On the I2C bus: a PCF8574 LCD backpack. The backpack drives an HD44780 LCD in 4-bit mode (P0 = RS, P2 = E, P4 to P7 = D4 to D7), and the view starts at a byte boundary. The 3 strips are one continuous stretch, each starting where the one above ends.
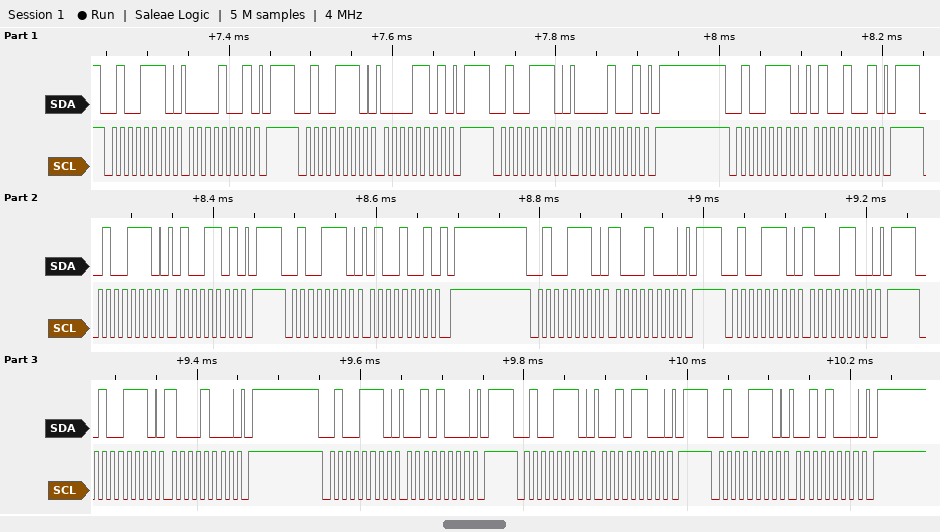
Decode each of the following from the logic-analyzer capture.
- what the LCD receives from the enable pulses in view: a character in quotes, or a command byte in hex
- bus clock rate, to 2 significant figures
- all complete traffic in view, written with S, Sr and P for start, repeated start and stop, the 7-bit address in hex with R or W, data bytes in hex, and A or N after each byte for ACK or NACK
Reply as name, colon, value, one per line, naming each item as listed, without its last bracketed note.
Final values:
what the LCD receives from the enable pulses in view: a character in quotes, or a command byte in hex: data 0x04 0x82
bus clock rate, to 2 significant figures: 100 kHz
all complete traffic in view, written with S, Sr and P for start, repeated start and stop, the 7-bit address in hex with R or W, data bytes in hex, and A or N after each byte for ACK or NACK: S 27W A 09 A P S 27W A 0D A P S 27W A 09 A P S 27W A 49 A P S 27W A 4D A P S 27W A 49 A P S 27W A 88 A P S 27W A 8C A P S 27W A 88 A P S 27W A 28 A P S 27W A 2C A P S 27W A 28 A P
